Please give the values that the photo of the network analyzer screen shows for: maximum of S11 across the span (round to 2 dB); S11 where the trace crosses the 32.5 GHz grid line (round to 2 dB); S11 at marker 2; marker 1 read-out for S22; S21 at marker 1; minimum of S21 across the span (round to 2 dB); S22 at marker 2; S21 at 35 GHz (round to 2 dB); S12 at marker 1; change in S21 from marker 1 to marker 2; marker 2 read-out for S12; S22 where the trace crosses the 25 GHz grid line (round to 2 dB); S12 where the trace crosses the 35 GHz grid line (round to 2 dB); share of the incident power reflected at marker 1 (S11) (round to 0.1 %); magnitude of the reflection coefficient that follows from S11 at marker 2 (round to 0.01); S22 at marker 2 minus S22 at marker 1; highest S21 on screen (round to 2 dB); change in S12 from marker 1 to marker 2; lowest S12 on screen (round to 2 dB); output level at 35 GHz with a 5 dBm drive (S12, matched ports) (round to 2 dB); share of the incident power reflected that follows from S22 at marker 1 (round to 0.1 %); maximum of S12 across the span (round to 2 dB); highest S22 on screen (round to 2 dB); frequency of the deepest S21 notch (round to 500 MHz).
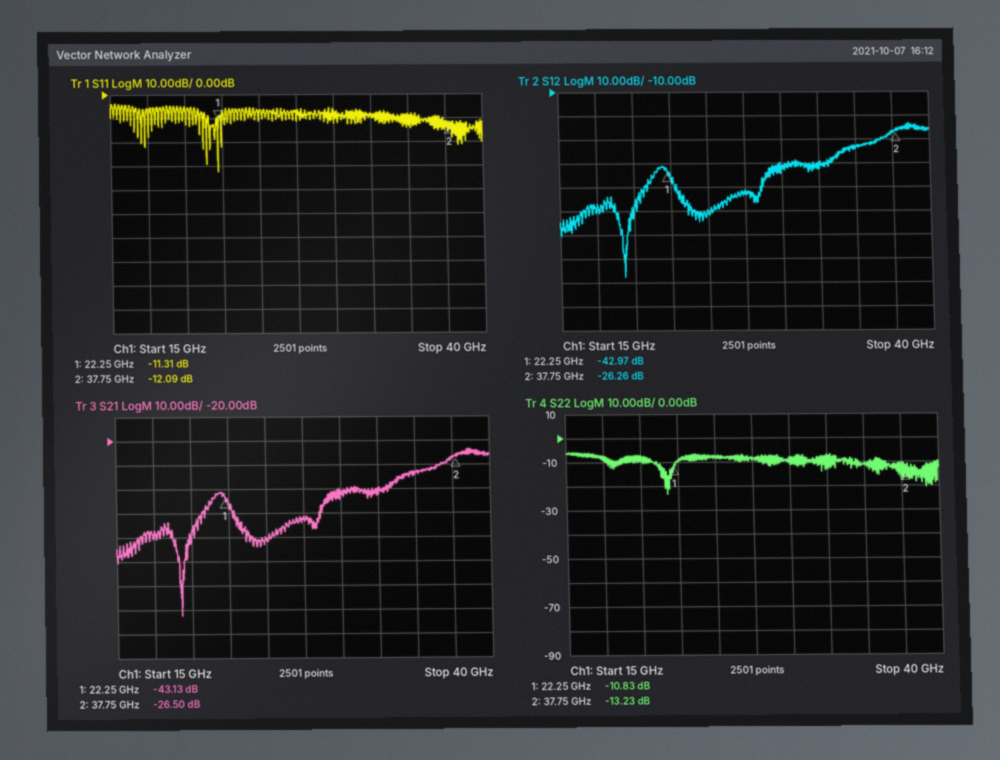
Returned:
-4 dB
-8 dB
-12.09 dB
-10.83 dB
-43.13 dB
-92 dB
-13.23 dB
-34 dB
-42.97 dB
16.63 dB
-26.26 dB
-8 dB
-34 dB
7.4 %
0.25
-2.40 dB
-24 dB
16.71 dB
-88 dB
-28 dBm
8.3 %
-24 dB
-6 dB
19.5 GHz
